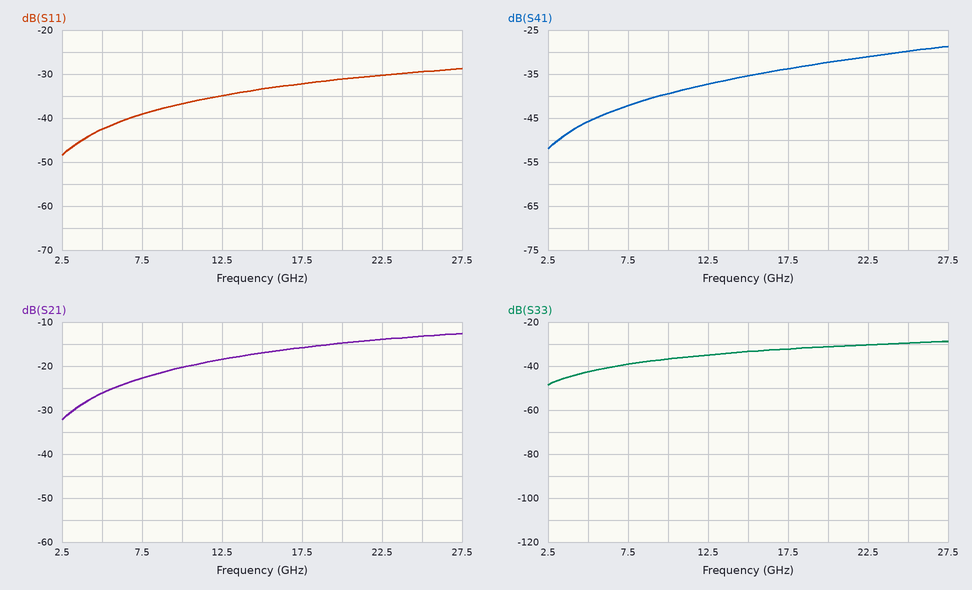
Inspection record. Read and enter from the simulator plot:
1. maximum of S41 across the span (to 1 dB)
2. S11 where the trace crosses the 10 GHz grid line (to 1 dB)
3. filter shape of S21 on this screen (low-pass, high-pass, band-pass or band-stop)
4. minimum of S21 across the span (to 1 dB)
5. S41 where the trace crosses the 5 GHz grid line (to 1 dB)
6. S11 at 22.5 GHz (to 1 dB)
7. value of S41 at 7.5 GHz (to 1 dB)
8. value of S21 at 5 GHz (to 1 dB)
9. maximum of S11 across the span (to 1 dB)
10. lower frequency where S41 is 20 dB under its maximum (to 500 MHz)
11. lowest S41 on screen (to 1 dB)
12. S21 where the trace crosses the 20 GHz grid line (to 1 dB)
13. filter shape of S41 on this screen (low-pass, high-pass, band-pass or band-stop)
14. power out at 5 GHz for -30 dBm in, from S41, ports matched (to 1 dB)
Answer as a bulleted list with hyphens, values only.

- -29 dB
- -37 dB
- high-pass
- -32 dB
- -46 dB
- -30 dB
- -42 dB
- -26 dB
- -29 dB
- 3.5 GHz
- -52 dB
- -15 dB
- high-pass
- -76 dBm
